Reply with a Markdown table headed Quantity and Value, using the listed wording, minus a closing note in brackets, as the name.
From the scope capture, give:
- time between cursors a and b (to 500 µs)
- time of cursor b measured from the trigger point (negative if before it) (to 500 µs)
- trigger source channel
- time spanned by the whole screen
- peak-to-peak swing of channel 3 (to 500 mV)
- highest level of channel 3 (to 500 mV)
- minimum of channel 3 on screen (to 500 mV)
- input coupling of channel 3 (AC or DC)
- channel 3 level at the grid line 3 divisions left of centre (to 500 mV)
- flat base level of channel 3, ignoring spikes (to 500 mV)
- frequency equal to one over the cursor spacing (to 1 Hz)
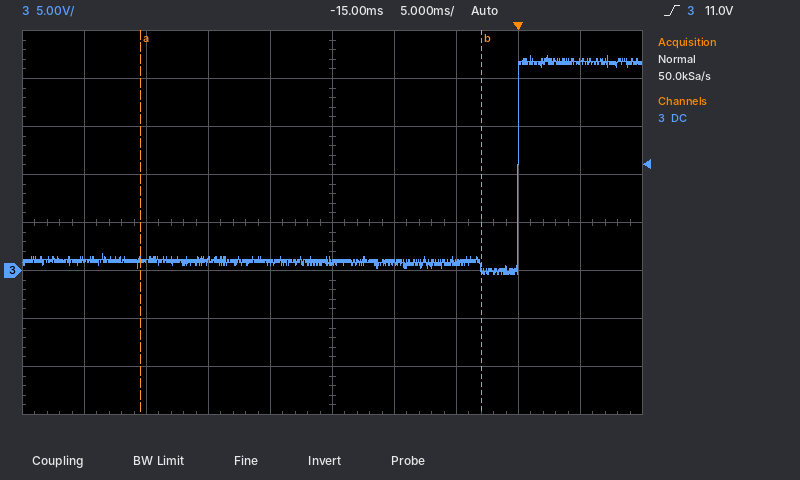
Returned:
| Quantity | Value |
|---|---|
| time between cursors a and b | 27.5 ms |
| time of cursor b measured from the trigger point (negative if before it) | -3.0 ms |
| trigger source channel | channel 3 |
| time spanned by the whole screen | 50 ms |
| peak-to-peak swing of channel 3 | 23.0 V |
| highest level of channel 3 | 22.5 V |
| minimum of channel 3 on screen | -500 mV |
| input coupling of channel 3 | DC |
| channel 3 level at the grid line 3 divisions left of centre | 1.0 V |
| flat base level of channel 3, ignoring spikes | 1.0 V |
| frequency equal to one over the cursor spacing | 36 Hz |
